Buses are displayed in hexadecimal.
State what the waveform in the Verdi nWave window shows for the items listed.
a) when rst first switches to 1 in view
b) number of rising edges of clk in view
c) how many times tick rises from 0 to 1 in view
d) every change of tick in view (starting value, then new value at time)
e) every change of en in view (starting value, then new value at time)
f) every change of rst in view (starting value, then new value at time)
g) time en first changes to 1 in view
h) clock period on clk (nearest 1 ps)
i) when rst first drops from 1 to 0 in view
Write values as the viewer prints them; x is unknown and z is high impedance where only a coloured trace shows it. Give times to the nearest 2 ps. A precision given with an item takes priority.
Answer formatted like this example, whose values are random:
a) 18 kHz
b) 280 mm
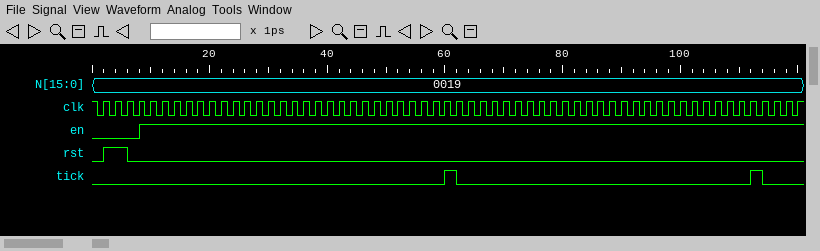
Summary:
a) 2 ps
b) 60
c) 2
d) 0, 1 at 60 ps, 0 at 62 ps, 1 at 112 ps, 0 at 114 ps
e) 0, 1 at 8 ps
f) 0, 1 at 2 ps, 0 at 6 ps
g) 8 ps
h) 2 ps
i) 6 ps
